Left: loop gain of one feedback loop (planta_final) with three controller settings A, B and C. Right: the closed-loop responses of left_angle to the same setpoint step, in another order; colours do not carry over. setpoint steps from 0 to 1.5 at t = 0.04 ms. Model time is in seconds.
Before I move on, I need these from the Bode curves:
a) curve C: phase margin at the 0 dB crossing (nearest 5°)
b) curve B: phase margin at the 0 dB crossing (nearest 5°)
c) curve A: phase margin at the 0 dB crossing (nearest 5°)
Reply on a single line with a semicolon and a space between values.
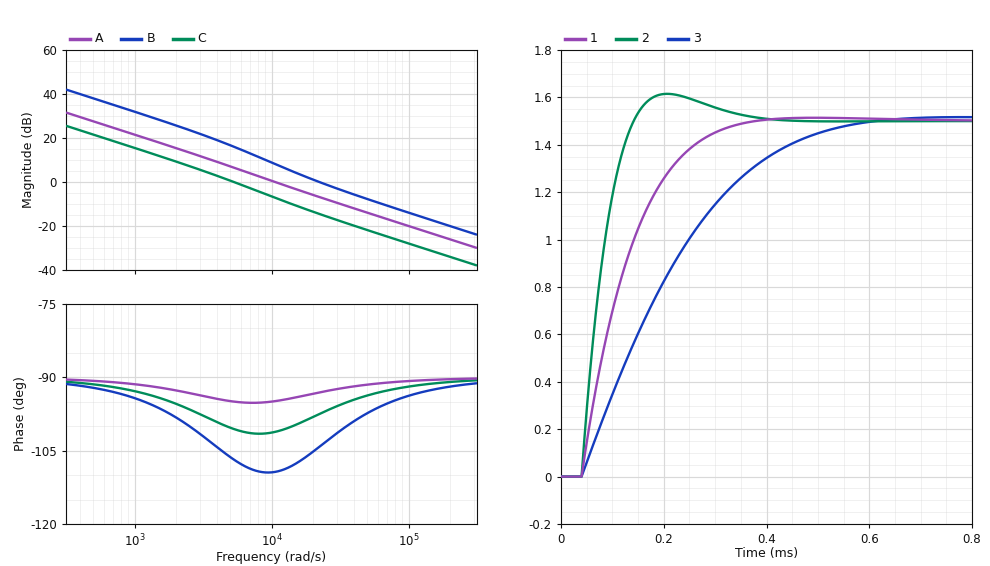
80°; 75°; 85°
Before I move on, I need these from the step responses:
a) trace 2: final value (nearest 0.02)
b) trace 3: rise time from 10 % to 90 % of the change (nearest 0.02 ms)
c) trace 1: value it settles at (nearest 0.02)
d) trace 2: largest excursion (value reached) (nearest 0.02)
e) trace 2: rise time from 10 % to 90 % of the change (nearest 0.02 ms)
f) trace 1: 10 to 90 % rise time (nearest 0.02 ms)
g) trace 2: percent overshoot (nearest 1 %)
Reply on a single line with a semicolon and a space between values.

1.50; 0.34 ms; 1.50; 1.62; 0.08 ms; 0.18 ms; 8 %
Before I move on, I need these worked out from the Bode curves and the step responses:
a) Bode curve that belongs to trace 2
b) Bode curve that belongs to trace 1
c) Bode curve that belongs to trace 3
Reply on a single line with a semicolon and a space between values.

B; A; C
